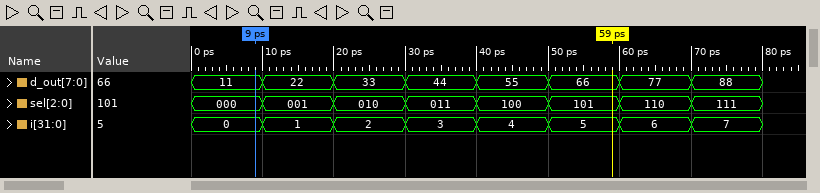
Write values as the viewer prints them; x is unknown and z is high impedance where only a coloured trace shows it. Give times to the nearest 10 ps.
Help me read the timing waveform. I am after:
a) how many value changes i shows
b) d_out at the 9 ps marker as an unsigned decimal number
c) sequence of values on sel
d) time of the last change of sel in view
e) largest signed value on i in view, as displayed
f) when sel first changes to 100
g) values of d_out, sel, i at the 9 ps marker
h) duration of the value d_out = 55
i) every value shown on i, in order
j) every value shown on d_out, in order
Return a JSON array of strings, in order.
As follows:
["7", "17", "000, 001, 010, 011, 100, 101, 110, 111", "70 ps", "7", "40 ps", "d_out=11, sel=000, i=0", "10 ps", "0, 1, 2, 3, 4, 5, 6, 7", "11, 22, 33, 44, 55, 66, 77, 88"]
